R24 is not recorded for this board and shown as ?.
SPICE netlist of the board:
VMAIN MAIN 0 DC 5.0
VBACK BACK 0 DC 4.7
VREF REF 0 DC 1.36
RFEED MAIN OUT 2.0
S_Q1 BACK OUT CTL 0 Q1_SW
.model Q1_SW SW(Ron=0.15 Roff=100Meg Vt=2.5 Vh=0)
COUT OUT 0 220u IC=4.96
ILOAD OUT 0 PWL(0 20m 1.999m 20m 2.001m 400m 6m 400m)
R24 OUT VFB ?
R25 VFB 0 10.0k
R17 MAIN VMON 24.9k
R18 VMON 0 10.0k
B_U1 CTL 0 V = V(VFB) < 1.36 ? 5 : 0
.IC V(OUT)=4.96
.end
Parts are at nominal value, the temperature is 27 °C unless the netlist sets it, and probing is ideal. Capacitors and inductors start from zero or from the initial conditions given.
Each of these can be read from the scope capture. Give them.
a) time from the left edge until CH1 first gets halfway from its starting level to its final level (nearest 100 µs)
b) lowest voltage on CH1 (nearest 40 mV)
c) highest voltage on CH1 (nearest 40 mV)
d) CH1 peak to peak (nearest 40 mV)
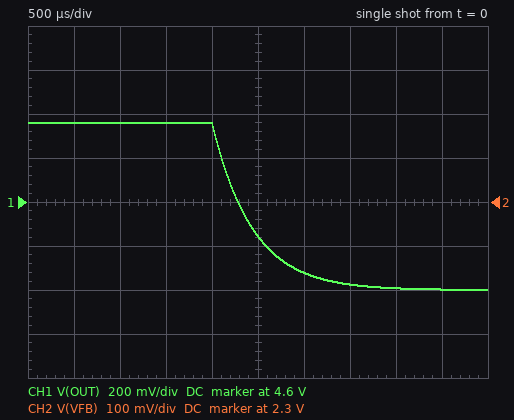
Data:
2.3 ms
4.20 V
4.96 V
760 mV
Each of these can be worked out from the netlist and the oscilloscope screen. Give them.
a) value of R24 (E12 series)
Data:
10 kΩ
